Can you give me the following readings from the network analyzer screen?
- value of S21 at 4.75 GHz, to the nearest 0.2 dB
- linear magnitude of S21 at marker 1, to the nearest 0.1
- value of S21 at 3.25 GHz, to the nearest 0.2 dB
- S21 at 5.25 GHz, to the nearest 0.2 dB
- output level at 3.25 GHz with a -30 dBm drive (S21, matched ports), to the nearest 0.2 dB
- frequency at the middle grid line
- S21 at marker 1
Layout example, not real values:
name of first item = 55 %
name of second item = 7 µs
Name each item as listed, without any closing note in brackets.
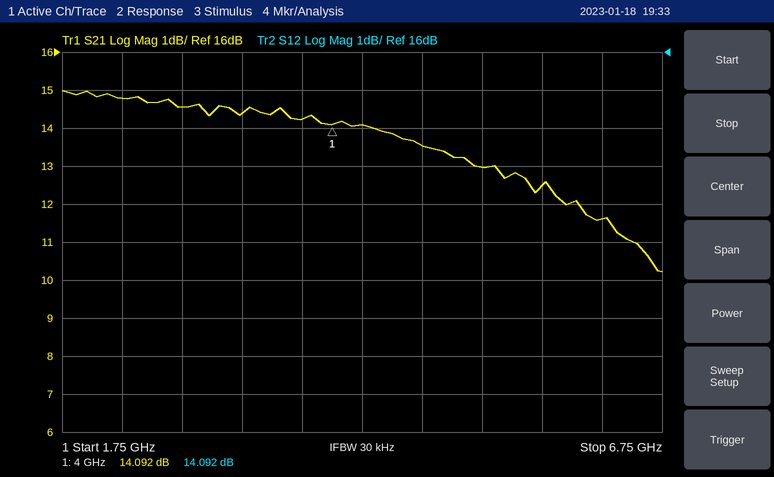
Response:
value of S21 at 4.75 GHz, to the nearest 0.2 dB = 13.6 dB
linear magnitude of S21 at marker 1, to the nearest 0.1 = 5.1
value of S21 at 3.25 GHz, to the nearest 0.2 dB = 14.4 dB
S21 at 5.25 GHz, to the nearest 0.2 dB = 13.0 dB
output level at 3.25 GHz with a -30 dBm drive (S21, matched ports), to the nearest 0.2 dB = -15.6 dBm
frequency at the middle grid line = 4.25 GHz
S21 at marker 1 = 14.092 dB
